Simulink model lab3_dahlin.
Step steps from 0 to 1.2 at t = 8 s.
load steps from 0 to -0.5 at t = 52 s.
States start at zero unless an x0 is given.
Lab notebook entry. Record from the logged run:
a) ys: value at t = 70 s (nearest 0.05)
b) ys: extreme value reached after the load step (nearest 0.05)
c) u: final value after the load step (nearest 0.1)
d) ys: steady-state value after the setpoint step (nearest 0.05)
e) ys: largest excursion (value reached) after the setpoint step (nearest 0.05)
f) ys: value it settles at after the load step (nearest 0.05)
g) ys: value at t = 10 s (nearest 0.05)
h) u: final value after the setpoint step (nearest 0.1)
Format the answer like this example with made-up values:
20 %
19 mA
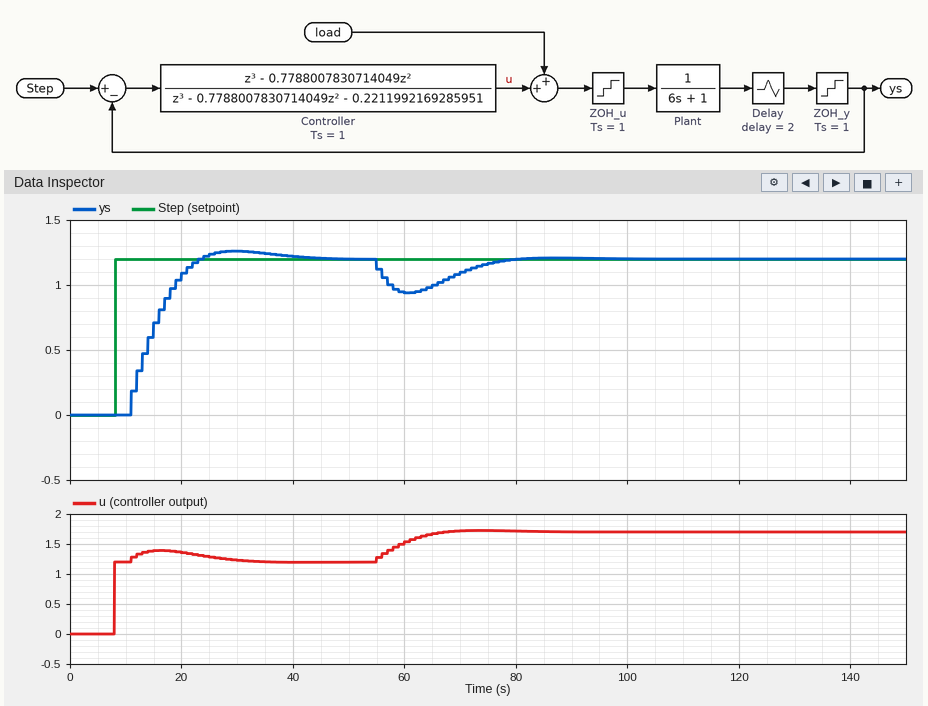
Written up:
1.10
0.95
1.7
1.20
1.25
1.20
0.00
1.2
